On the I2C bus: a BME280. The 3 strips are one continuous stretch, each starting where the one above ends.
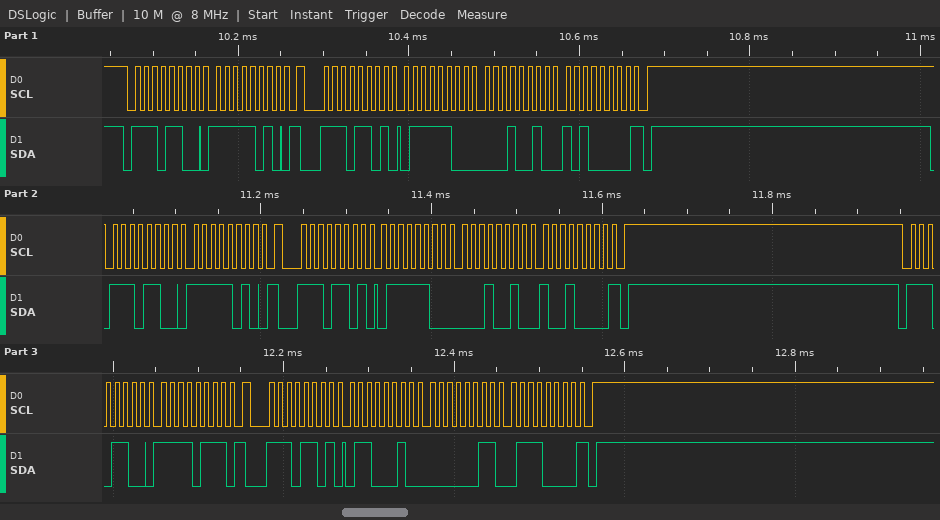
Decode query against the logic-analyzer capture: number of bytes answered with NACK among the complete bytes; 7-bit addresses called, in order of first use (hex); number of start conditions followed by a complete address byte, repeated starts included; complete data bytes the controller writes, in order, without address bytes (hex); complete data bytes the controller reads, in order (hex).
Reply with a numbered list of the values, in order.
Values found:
1. 3
2. 0x76
3. 6
4. FA FA F7
5. 7C 12 A0 7C 12 90 62 03 70
